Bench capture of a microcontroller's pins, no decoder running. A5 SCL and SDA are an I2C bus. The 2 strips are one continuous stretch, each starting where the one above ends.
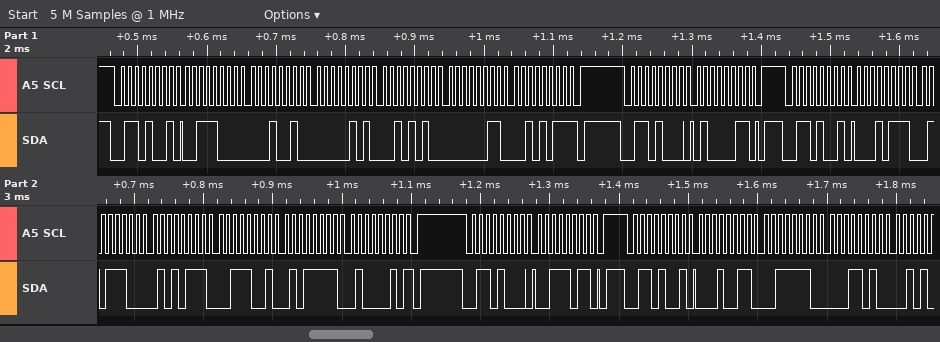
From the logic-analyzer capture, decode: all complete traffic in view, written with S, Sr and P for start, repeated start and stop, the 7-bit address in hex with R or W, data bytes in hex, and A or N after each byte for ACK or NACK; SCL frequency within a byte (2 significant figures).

S 34R A 38 A 12 A 05 A 2A A 03 A 2B N P S 34W A 43 A P S 34R A 17 A 5C A 57 A 39 A 5F A 42 N P S 34W A 3B A P S 34R A 13 A 3E A 1A A
100 kHz
